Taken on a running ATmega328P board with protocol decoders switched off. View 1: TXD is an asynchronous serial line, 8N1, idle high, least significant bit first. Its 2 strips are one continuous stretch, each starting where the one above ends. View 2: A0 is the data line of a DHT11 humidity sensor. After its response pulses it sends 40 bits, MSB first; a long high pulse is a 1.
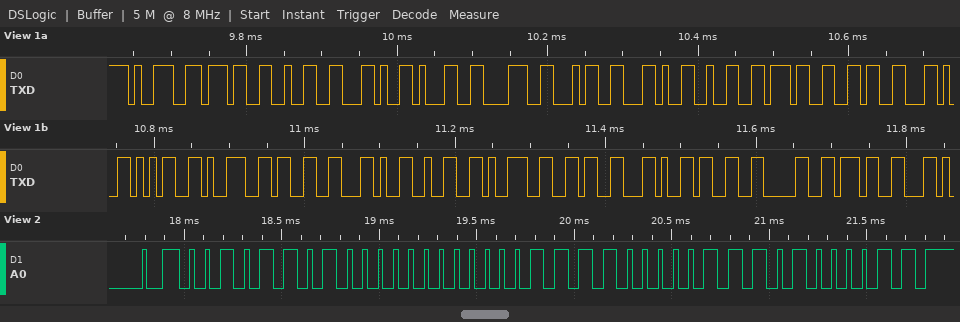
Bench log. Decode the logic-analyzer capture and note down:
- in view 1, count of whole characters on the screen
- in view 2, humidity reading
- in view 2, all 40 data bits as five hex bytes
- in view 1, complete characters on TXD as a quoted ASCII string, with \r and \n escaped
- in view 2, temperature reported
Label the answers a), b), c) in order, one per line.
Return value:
a) 23
b) 45 %
c) 2D 00 0F 07 43
d) "972,184,276,593,296,307"
e) 15.7 °C
